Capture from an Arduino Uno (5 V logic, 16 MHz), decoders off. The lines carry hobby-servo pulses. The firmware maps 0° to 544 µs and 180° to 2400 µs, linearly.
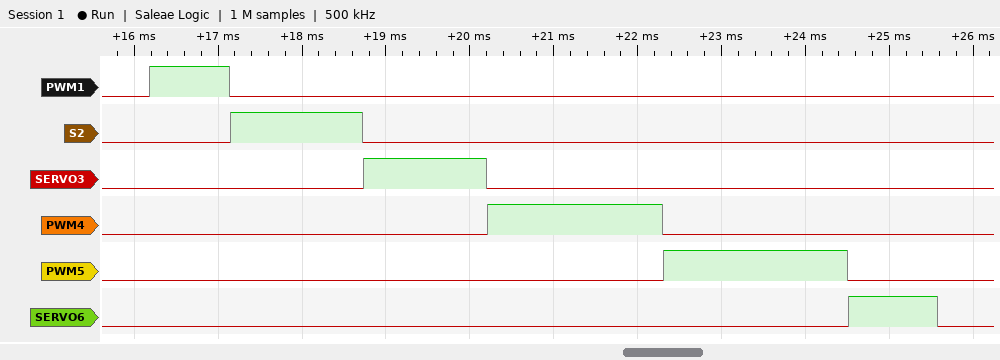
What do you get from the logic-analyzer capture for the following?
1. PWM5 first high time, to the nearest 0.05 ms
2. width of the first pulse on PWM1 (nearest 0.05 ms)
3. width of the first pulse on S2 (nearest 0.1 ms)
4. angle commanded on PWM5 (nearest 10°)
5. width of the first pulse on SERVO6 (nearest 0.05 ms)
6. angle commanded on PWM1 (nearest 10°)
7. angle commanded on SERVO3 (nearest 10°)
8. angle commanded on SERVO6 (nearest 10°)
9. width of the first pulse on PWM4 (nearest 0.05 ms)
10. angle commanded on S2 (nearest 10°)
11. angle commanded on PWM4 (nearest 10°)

2.20 ms
0.95 ms
1.6 ms
160°
1.05 ms
40°
90°
50°
2.10 ms
100°
150°
